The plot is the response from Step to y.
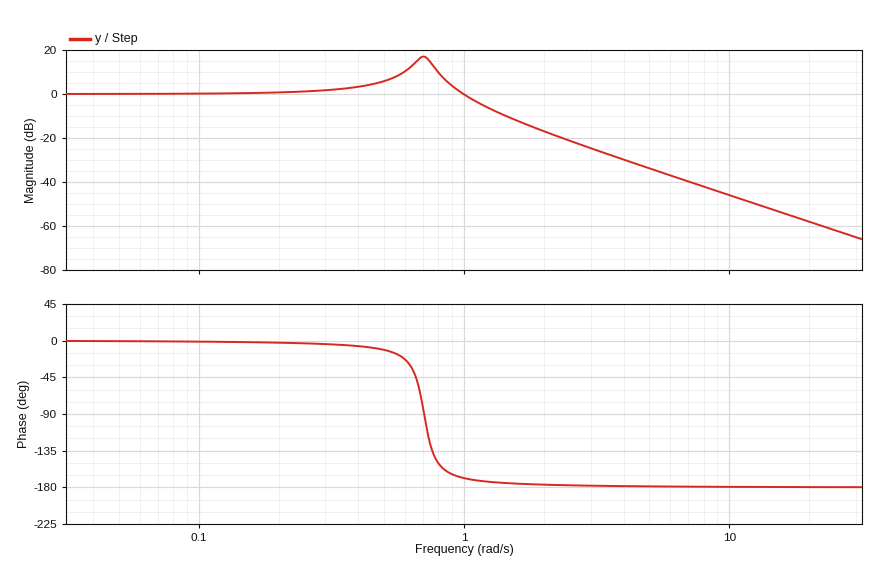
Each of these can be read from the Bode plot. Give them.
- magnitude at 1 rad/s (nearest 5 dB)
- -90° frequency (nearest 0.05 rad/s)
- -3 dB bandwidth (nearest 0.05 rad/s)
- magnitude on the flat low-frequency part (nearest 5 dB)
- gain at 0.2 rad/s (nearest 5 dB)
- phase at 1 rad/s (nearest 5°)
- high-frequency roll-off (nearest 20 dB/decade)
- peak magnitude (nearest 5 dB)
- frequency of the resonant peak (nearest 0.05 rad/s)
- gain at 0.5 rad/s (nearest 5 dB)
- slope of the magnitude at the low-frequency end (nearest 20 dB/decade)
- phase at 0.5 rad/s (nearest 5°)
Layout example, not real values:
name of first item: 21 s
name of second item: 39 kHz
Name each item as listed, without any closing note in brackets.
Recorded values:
magnitude at 1 rad/s: 0 dB
-90° frequency: 0.70 rad/s
-3 dB bandwidth: 1.10 rad/s
magnitude on the flat low-frequency part: 0 dB
gain at 0.2 rad/s: 0 dB
phase at 1 rad/s: -170°
high-frequency roll-off: -40 dB/decade
peak magnitude: 15 dB
frequency of the resonant peak: 0.70 rad/s
gain at 0.5 rad/s: 5 dB
slope of the magnitude at the low-frequency end: 0 dB/decade
phase at 0.5 rad/s: -10°
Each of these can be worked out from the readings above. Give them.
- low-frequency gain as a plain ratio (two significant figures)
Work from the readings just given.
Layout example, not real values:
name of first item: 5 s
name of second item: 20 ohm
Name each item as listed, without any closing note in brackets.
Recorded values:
low-frequency gain as a plain ratio: 1.0
